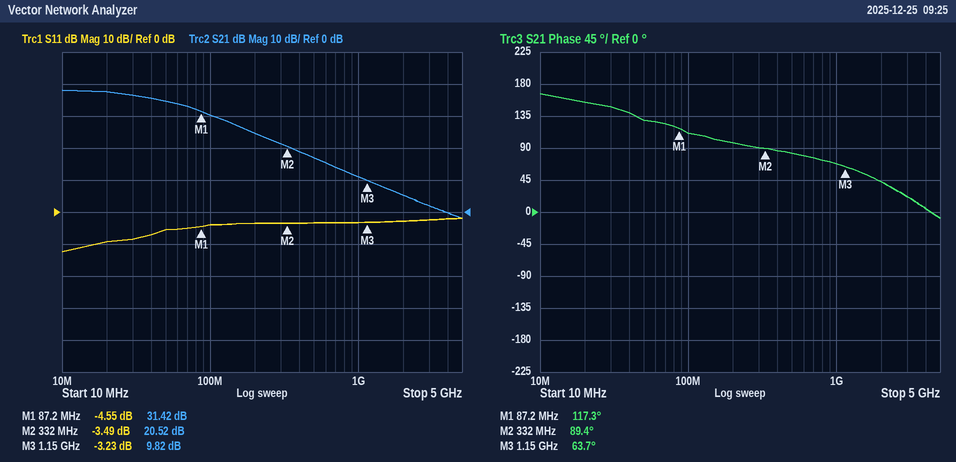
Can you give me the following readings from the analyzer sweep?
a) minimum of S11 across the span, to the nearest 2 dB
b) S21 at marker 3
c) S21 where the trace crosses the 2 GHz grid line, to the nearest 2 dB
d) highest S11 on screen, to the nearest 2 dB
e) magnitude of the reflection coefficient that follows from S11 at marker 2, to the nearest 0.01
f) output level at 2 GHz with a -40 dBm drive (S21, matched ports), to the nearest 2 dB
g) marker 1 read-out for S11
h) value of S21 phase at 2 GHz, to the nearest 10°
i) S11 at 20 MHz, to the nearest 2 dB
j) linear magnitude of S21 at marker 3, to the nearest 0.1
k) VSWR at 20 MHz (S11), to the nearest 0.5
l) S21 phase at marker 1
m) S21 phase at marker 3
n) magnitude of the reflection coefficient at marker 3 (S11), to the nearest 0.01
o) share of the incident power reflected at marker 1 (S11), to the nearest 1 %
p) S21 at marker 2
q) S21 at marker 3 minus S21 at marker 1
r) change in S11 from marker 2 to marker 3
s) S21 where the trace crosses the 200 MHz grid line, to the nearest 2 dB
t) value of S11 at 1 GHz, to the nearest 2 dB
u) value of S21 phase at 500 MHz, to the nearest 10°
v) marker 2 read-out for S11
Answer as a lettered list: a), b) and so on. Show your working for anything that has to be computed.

a) -12 dB
b) 9.82 dB
c) 6 dB
d) -2 dB
e) 10^(-3.49/20) ≈ 0.67
f) -40 dBm + (6 dB) = -34 dBm
g) -4.55 dB
h) 40°
i) -10 dB
j) 10^(9.82/20) ≈ 3.1
k) |Γ| = 10^(-10/20) = 0.3162; VSWR = (1 + 0.3162)/(1 − 0.3162) ≈ 1.92, so 2.0 to the nearest 0.5
l) 117.3°
m) 63.7°
n) 10^(-3.23/20) ≈ 0.69
o) 10^(-4.55/10) ≈ 35 %
p) 20.52 dB
q) 9.82 − (31.42) = -21.60 dB
r) -3.23 − (-3.49) = 0.26 dB
s) 24 dB
t) -4 dB
u) 80°
v) -3.49 dB
